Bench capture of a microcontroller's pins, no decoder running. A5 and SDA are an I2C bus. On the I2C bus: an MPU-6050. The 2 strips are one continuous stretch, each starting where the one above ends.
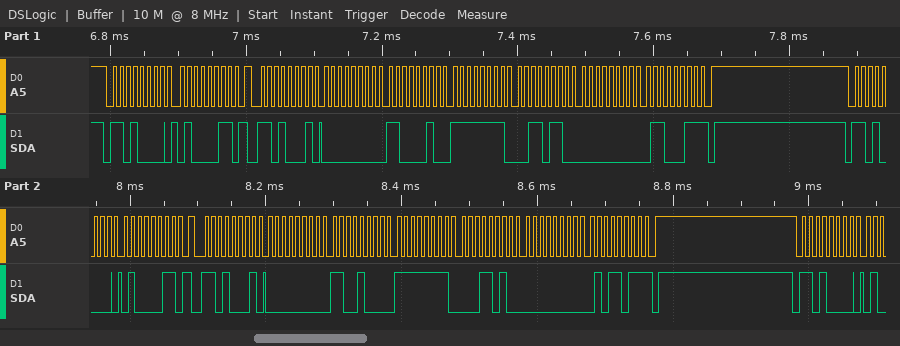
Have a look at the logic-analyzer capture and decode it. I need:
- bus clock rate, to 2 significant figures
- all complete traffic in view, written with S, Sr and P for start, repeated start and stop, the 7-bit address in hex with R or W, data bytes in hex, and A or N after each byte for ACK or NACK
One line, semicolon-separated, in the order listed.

100 kHz; S 68W A 43 A Sr 68R A 00 A C2 A FF A 36 A 00 A 63 N P S 68W A 43 A Sr 68R A 00 A C8 A FF A 1A A 00 A 5B N P S 68W A
